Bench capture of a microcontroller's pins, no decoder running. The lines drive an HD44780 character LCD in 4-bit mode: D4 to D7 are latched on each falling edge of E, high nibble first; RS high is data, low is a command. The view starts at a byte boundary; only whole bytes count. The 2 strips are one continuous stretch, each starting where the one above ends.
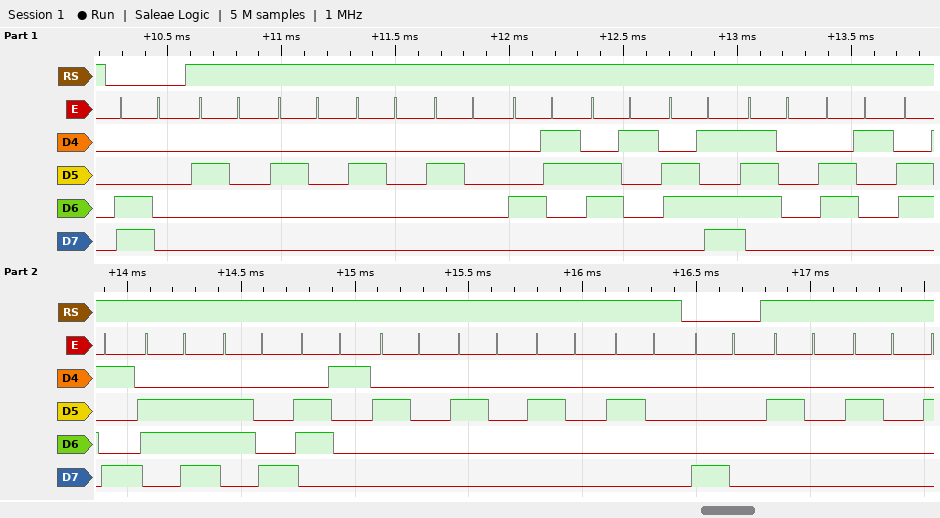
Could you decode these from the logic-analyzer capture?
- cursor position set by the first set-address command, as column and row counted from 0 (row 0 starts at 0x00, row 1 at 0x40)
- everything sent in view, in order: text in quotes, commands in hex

column 0, row 1
0xC0 "    Campainha    " 0x80 "  "
